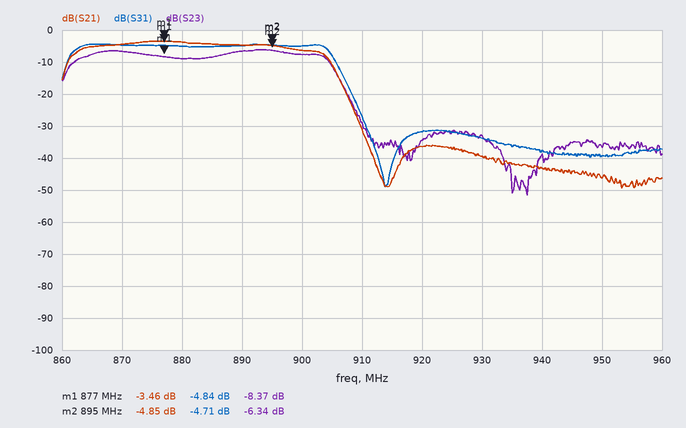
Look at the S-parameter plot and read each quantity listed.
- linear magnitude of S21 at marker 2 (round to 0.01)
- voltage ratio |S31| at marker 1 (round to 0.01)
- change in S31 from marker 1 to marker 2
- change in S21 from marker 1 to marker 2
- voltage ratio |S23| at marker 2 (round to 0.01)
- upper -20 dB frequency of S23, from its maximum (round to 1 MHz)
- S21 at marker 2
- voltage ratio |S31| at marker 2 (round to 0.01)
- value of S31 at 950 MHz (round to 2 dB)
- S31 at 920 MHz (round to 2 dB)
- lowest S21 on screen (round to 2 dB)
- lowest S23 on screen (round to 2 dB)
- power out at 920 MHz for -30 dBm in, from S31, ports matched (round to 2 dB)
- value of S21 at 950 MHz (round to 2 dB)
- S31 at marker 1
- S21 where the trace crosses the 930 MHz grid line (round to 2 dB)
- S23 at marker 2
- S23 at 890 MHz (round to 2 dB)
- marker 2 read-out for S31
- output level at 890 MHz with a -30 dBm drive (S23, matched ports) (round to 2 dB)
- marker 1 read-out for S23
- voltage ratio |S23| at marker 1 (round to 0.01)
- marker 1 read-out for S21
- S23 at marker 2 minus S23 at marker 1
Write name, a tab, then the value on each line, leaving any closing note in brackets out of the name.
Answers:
linear magnitude of S21 at marker 2	0.57
voltage ratio |S31| at marker 1	0.57
change in S31 from marker 1 to marker 2	0.13 dB
change in S21 from marker 1 to marker 2	-1.39 dB
voltage ratio |S23| at marker 2	0.48
upper -20 dB frequency of S23, from its maximum	909 MHz
S21 at marker 2	-4.85 dB
voltage ratio |S31| at marker 2	0.58
value of S31 at 950 MHz	-40 dB
S31 at 920 MHz	-32 dB
lowest S21 on screen	-50 dB
lowest S23 on screen	-52 dB
power out at 920 MHz for -30 dBm in, from S31, ports matched	-62 dBm
value of S21 at 950 MHz	-46 dB
S31 at marker 1	-4.84 dB
S21 where the trace crosses the 930 MHz grid line	-40 dB
S23 at marker 2	-6.34 dB
S23 at 890 MHz	-6 dB
marker 2 read-out for S31	-4.71 dB
output level at 890 MHz with a -30 dBm drive (S23, matched ports)	-36 dBm
marker 1 read-out for S23	-8.37 dB
voltage ratio |S23| at marker 1	0.38
marker 1 read-out for S21	-3.46 dB
S23 at marker 2 minus S23 at marker 1	2.03 dB
